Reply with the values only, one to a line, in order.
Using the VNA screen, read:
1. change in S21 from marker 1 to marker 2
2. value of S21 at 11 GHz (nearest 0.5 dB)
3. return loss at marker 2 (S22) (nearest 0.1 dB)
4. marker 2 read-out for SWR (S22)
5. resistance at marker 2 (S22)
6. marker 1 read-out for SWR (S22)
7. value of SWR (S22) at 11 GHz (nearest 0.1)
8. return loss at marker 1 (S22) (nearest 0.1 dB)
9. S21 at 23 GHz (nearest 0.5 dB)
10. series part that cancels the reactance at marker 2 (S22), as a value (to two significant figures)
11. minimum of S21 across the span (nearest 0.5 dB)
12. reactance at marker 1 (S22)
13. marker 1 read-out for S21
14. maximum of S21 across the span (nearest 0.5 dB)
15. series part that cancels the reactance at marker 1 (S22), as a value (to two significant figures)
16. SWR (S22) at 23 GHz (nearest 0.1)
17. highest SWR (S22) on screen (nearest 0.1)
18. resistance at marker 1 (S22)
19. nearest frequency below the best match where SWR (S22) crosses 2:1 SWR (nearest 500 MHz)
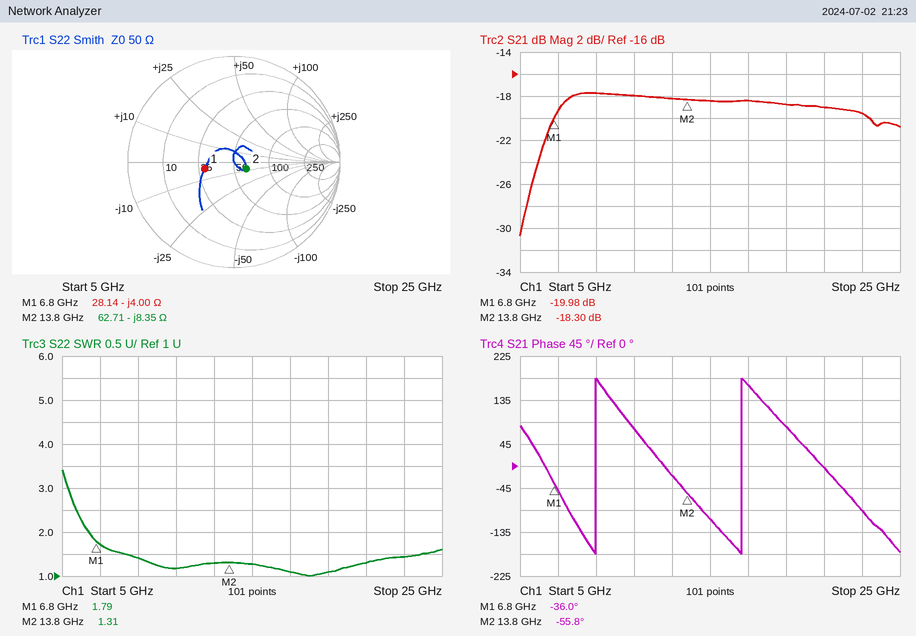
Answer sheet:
1.68 dB
-18.0 dB
17.4 dB
1.31
62.71 Ω
1.79
1.2
10.9 dB
-19.5 dB
96 pH
-30.5 dB
-4.00 Ω
-19.98 dB
-17.5 dB
94 pH
1.4
3.4
28.14 Ω
6.5 GHz
